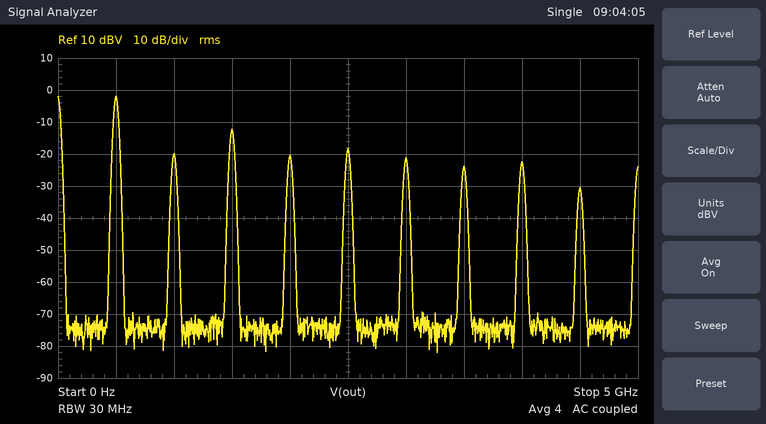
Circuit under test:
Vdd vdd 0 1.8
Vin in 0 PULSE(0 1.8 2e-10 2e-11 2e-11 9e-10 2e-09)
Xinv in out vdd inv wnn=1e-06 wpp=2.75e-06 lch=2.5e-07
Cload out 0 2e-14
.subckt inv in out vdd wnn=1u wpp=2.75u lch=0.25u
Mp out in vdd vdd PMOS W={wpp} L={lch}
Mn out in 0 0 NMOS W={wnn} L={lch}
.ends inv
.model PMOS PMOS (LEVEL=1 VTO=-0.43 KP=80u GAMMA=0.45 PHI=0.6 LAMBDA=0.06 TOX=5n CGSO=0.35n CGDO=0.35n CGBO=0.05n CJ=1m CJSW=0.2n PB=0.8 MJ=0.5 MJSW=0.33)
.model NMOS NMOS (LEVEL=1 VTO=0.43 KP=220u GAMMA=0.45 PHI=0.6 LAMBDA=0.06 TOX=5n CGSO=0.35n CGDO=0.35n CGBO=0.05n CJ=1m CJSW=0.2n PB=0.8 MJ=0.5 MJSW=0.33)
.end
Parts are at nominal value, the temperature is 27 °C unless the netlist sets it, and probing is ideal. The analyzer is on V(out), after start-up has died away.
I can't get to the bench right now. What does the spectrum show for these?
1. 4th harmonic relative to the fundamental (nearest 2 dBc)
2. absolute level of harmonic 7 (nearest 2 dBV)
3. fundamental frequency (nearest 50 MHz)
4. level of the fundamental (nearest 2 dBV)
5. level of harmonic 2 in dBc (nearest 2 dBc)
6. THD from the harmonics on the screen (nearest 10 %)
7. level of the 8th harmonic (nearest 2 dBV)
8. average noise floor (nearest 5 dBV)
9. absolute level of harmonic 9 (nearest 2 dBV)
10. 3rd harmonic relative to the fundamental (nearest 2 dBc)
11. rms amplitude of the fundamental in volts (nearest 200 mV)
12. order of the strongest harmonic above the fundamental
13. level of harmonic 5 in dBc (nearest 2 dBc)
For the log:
-18 dBc
-24 dBV
500 MHz
-2 dBV
-18 dBc
40 %
-22 dBV
-75 dBV
-30 dBV
-10 dBc
800 mV
3
-16 dBc
